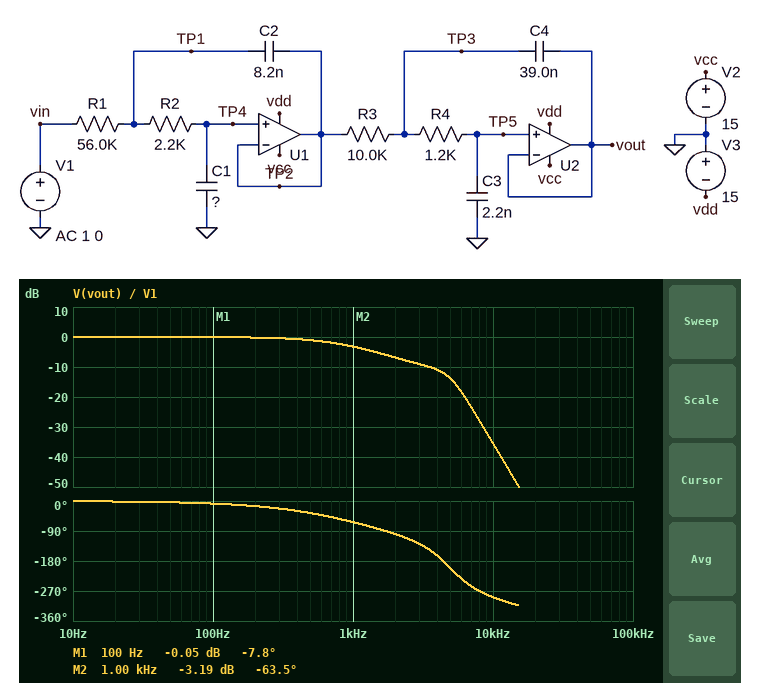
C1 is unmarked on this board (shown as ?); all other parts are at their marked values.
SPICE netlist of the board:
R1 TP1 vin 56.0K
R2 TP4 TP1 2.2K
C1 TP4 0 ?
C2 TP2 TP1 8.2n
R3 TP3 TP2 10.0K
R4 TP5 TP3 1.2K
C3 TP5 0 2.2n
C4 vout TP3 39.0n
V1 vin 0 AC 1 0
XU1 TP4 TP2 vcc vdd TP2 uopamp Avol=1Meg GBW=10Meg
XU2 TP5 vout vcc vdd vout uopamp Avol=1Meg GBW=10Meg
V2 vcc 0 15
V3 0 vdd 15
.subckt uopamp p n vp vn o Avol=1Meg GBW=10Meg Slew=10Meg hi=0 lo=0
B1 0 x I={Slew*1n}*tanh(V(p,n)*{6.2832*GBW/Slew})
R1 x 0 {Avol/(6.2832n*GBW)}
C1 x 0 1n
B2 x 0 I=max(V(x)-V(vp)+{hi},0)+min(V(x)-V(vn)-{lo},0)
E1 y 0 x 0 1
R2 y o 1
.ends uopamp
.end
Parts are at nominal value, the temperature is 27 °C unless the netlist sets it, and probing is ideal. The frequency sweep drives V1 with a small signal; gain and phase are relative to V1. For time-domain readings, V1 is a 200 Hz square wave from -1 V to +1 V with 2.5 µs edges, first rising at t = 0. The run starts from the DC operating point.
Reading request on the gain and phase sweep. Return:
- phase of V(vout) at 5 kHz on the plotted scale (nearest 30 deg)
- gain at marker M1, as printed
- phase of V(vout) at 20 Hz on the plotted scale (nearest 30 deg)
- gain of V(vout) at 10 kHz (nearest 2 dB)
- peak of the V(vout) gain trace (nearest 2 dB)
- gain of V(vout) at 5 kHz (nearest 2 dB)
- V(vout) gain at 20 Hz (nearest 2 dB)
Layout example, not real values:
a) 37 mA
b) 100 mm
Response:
a) -210 deg
b) -0.05 dB
c) 0 deg
d) -36 dB
e) 0 dB
f) -14 dB
g) 0 dB
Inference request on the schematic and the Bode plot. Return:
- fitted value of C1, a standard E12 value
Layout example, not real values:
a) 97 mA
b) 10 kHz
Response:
a) 3.3 nF
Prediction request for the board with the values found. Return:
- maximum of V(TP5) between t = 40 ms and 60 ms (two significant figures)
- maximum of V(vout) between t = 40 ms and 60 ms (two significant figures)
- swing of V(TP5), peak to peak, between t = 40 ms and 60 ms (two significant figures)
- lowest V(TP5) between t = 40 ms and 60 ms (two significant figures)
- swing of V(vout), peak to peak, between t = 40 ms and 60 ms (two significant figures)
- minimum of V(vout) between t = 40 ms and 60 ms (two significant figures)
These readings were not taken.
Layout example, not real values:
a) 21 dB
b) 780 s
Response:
a) 1.0 V
b) 1.0 V
c) 2.0 V
d) -1.0 V
e) 2.0 V
f) -1.0 V
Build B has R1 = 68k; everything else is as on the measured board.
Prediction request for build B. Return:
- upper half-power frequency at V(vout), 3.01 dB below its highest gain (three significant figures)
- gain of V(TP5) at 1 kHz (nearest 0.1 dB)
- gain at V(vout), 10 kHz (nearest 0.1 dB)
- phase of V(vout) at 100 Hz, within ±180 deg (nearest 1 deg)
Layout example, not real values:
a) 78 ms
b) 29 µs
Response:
a) 768 Hz
b) -4.3 dB
c) -37.2 dB
d) -9 deg
